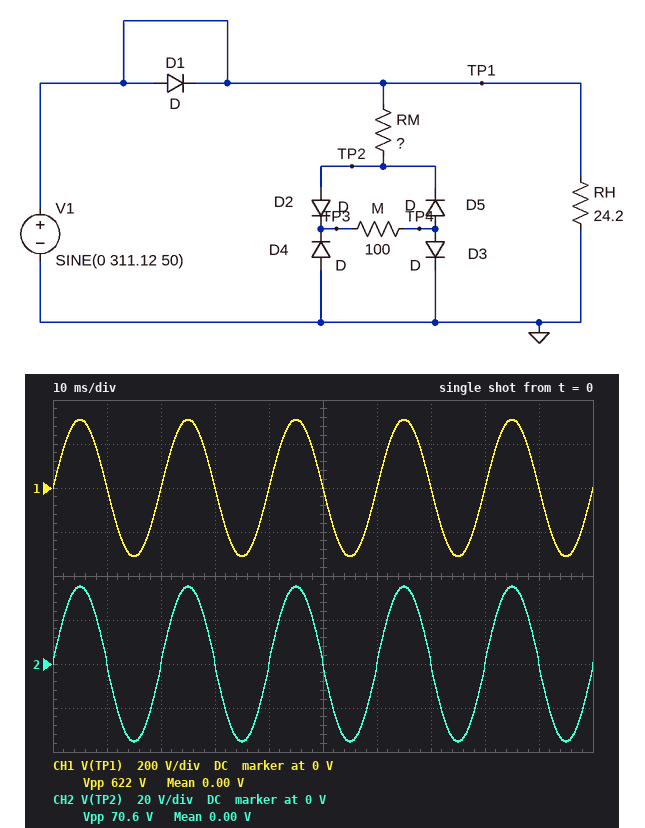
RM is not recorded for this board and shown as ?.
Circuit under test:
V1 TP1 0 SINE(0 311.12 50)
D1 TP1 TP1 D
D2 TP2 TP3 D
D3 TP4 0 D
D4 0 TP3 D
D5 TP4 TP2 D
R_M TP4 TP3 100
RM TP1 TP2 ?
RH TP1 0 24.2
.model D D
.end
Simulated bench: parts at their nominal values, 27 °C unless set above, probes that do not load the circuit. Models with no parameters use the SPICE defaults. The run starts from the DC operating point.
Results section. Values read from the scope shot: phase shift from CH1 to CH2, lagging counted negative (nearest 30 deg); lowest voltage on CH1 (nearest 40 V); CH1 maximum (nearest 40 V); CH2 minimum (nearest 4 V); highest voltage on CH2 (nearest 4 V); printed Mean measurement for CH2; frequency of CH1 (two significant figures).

0 deg
-320 V
320 V
-36 V
36 V
0.00 V
50 Hz
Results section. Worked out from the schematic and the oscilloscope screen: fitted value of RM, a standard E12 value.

820 Ω
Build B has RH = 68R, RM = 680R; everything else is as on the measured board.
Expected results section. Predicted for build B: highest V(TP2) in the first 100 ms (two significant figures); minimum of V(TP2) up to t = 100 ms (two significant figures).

41 V
-41 V
